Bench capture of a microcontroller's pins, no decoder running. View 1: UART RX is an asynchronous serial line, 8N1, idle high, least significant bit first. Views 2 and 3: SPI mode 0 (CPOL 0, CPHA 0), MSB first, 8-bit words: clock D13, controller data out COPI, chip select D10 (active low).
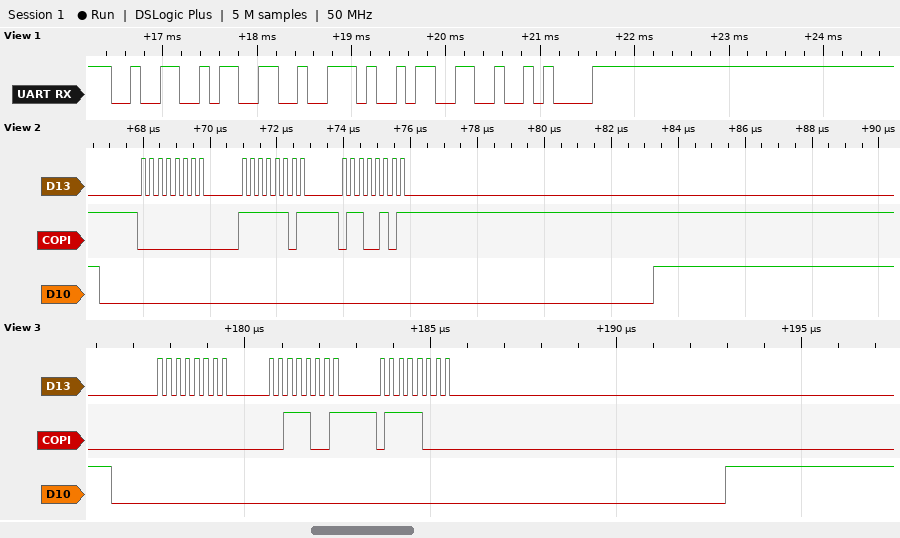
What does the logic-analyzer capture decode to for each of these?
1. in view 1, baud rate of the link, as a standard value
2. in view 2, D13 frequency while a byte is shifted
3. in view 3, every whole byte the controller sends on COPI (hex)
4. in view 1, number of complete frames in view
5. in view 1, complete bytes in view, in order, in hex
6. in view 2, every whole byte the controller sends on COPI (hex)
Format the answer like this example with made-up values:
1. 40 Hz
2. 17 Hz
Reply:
1. 9600 baud
2. 4 MHz
3. 0x00 0x39 0x78
4. 5
5. 0x32 0x33 0x2E 0x33 0x0A
6. 00 FD 65
